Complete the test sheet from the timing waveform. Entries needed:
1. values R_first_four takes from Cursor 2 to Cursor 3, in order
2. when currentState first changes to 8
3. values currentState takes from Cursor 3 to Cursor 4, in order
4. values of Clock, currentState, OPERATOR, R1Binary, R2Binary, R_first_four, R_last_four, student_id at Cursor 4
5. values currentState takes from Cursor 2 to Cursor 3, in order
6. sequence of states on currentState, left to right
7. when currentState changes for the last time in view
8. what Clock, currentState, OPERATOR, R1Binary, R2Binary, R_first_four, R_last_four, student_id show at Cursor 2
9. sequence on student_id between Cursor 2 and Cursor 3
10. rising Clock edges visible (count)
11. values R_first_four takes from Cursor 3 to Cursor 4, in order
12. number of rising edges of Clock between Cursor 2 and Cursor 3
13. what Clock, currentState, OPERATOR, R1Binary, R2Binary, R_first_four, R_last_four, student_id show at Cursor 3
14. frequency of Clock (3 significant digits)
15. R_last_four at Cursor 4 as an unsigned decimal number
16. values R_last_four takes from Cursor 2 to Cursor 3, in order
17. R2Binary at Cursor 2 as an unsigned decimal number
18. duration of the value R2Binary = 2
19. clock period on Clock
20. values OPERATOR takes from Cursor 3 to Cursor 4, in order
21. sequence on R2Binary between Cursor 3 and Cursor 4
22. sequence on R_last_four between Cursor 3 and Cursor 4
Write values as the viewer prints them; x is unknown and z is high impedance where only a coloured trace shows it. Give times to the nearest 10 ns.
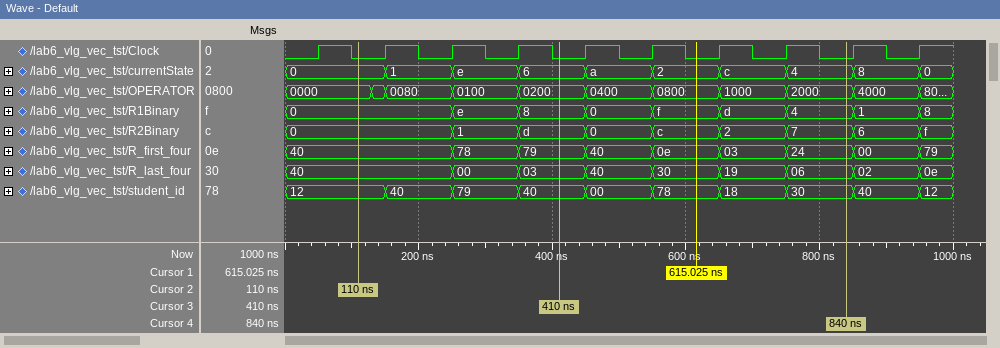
40, 78, 79
850 ns
6, a, 2, c, 4
Clock=0, currentState=4, OPERATOR=2000, R1Binary=4, R2Binary=7, R_first_four=24, R_last_four=06, student_id=30
0, 1, e, 6
0, 1, e, 6, a, 2, c, 4, 8, 0
950 ns
Clock=0, currentState=0, OPERATOR=0000, R1Binary=0, R2Binary=0, R_first_four=40, R_last_four=40, student_id=12
12, 40, 79, 40
10
79, 40, 0e, 03, 24
3
Clock=0, currentState=6, OPERATOR=0200, R1Binary=8, R2Binary=d, R_first_four=79, R_last_four=03, student_id=40
10.0 MHz
6
40, 00, 03
0
100 ns
100 ns
0200, 0400, 0800, 1000, 2000
d, 0, c, 2, 7
03, 40, 30, 19, 06
